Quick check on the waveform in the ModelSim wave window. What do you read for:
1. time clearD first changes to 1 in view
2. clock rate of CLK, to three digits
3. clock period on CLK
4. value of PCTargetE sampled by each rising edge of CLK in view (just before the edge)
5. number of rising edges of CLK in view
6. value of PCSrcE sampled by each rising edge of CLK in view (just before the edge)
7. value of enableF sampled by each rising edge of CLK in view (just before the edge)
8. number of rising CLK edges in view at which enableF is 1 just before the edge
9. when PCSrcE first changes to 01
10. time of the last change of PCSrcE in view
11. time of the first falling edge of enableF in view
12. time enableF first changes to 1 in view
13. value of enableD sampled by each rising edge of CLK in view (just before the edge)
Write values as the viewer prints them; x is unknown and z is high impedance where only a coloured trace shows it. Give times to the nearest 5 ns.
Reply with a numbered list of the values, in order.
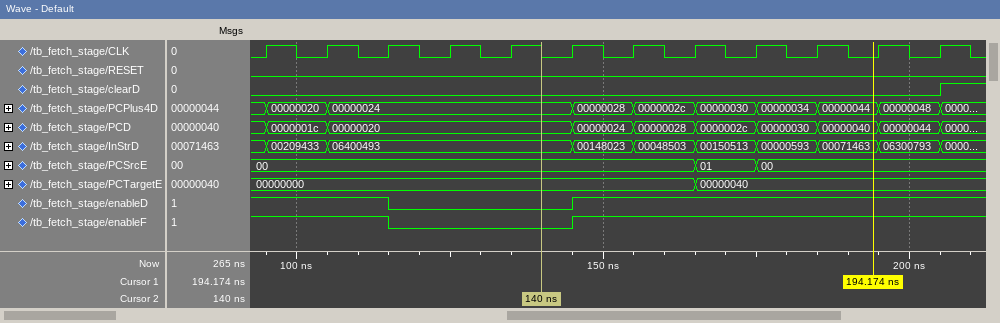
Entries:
1. 205 ns
2. 100 MHz
3. 10 ns
4. 00000000, 00000000, 00000000, 00000000, 00000000, 00000000, 00000000, 00000000, 00000040, 00000040, 00000040, 00000040
5. 12
6. 00, 00, 00, 00, 00, 00, 00, 00, 01, 00, 00, 00
7. 1 1 1 0 0 0 1 1 1 1 1 1
8. 9
9. 165 ns
10. 175 ns
11. 115 ns
12. 145 ns
13. 1 1 1 0 0 0 1 1 1 1 1 1
